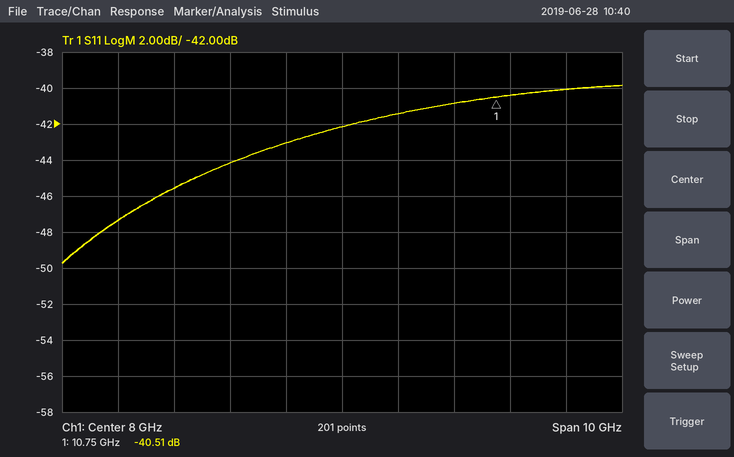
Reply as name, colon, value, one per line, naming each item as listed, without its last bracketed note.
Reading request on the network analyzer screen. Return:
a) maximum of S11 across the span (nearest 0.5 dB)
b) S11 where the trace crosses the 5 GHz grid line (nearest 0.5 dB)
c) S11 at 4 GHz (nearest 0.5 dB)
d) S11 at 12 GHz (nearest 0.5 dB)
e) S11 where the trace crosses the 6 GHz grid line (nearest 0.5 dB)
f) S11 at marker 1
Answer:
maximum of S11 across the span: -40.0 dB
S11 where the trace crosses the 5 GHz grid line: -45.5 dB
S11 at 4 GHz: -47.5 dB
S11 at 12 GHz: -40.0 dB
S11 where the trace crosses the 6 GHz grid line: -44.0 dB
S11 at marker 1: -40.51 dB
